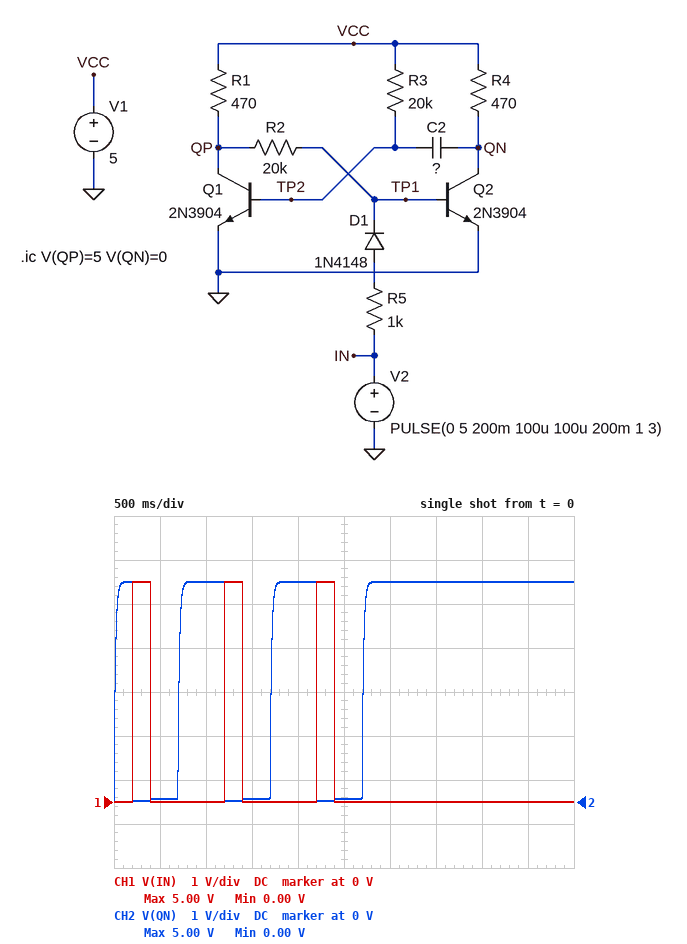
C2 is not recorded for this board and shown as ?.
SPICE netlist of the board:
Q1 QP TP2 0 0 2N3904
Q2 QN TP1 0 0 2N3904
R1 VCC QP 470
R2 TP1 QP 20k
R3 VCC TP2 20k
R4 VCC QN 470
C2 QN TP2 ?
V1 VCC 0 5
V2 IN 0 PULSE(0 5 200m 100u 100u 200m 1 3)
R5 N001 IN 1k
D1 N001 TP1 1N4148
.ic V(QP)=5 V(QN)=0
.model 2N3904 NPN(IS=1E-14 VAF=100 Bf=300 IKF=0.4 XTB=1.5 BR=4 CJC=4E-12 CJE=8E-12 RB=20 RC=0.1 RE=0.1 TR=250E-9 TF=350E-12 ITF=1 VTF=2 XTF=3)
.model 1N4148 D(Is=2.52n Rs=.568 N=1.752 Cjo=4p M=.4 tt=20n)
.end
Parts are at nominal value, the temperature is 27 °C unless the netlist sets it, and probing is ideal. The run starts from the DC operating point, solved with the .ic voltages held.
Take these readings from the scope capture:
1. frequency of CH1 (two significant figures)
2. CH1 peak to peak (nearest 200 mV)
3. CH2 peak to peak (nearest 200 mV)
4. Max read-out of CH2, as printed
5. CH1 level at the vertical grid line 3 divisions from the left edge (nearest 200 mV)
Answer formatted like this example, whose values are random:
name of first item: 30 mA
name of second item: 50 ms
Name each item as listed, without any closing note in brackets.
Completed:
frequency of CH1: 1.0 Hz
CH1 peak to peak: 5.0 V
CH2 peak to peak: 5.0 V
Max read-out of CH2, as printed: 5.00 V
CH1 level at the vertical grid line 3 divisions from the left edge: 0 V
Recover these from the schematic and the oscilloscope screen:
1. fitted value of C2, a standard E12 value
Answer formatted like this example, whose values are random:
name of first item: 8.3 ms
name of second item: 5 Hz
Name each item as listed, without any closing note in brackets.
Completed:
fitted value of C2, a standard E12 value: 33 µF
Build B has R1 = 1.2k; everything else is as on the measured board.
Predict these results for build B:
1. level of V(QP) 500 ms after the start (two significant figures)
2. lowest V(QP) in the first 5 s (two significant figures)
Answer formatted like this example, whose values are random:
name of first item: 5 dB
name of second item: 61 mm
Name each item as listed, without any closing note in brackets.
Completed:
level of V(QP) 500 ms after the start: 4.8 V
lowest V(QP) in the first 5 s: 11 mV
